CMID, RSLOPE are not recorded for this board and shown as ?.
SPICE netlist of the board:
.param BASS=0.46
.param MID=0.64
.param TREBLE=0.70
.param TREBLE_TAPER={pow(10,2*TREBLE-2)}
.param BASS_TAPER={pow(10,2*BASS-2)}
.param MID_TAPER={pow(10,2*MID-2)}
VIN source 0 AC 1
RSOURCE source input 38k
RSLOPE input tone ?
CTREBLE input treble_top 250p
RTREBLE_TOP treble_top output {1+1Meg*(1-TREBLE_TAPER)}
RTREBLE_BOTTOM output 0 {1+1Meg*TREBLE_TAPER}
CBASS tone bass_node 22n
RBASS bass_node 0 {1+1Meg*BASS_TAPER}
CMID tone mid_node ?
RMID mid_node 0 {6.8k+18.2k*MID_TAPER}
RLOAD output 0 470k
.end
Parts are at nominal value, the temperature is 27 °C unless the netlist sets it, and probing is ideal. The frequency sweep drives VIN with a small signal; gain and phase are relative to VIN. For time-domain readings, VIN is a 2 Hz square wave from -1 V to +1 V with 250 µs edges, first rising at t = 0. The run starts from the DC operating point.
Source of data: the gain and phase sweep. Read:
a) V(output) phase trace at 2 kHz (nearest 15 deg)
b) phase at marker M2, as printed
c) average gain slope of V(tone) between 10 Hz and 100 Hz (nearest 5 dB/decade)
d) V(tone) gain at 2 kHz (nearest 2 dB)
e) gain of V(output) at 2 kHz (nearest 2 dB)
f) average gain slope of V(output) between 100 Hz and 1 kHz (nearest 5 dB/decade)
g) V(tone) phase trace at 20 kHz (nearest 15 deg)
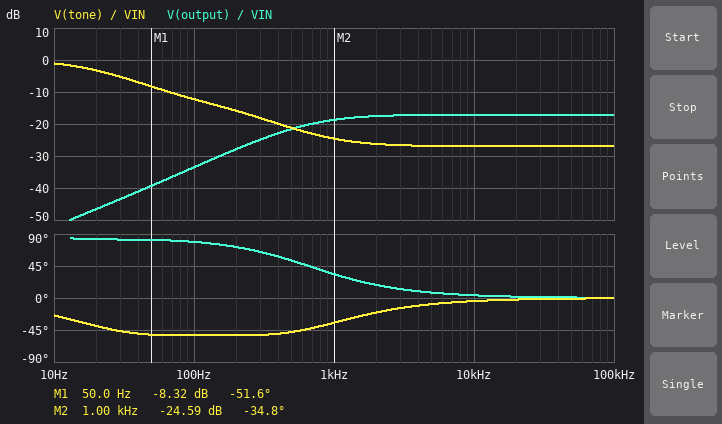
15 deg
-34.8 deg
-10 dB/decade
-26 dB
-18 dB
15 dB/decade
0 deg
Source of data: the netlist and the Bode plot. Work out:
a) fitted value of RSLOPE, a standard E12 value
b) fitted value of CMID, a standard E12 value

150 kΩ
18 nF
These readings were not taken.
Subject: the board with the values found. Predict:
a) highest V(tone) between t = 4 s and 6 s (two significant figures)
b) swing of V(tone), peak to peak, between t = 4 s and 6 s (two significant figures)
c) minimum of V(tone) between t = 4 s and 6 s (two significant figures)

1.0 V
2.0 V
-1.0 V
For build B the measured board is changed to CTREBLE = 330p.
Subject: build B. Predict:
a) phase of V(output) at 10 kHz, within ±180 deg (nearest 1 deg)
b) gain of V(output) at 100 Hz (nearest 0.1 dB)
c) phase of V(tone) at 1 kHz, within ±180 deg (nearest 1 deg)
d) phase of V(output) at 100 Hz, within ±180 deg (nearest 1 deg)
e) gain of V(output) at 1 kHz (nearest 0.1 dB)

3 deg
-31.2 dB
-35 deg
76 deg
-18.1 dB
